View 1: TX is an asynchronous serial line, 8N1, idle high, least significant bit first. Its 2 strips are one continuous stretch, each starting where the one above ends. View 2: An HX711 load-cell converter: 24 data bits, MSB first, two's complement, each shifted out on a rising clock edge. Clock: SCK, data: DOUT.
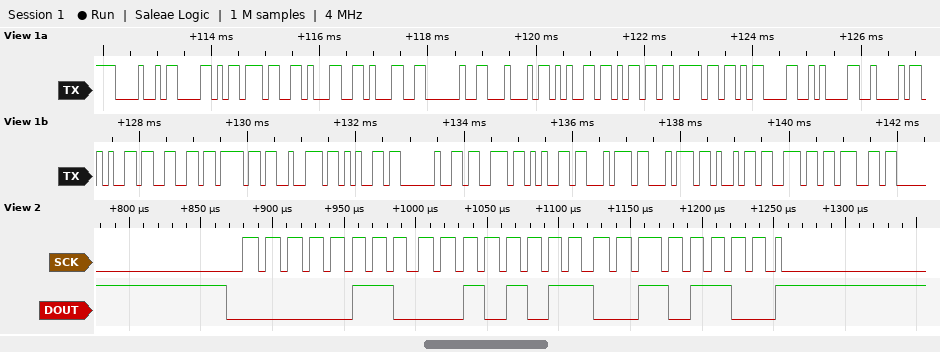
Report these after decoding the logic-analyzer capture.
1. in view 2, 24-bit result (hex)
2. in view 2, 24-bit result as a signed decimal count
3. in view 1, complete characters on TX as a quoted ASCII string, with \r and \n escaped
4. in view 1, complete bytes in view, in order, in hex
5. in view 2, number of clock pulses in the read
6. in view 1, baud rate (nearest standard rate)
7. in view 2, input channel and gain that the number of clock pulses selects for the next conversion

0x062B2C
404268
"HX711 Demo\r\nBefore setting"
0x48 0x58 0x37 0x31 0x31 0x20 0x44 0x65 0x6D 0x6F 0x0D 0x0A 0x42 0x65 0x66 0x6F 0x72 0x65 0x20 0x73 0x65 0x74 0x74 0x69 0x6E 0x67
25
9600 baud
channel A, gain 128
